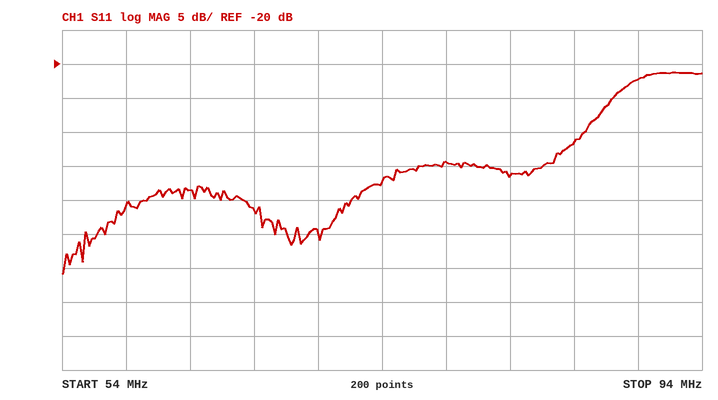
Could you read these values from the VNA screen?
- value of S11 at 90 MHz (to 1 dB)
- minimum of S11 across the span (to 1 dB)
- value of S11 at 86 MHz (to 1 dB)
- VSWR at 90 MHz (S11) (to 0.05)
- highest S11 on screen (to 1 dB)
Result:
-22 dB
-51 dB
-32 dB
1.15
-21 dB
